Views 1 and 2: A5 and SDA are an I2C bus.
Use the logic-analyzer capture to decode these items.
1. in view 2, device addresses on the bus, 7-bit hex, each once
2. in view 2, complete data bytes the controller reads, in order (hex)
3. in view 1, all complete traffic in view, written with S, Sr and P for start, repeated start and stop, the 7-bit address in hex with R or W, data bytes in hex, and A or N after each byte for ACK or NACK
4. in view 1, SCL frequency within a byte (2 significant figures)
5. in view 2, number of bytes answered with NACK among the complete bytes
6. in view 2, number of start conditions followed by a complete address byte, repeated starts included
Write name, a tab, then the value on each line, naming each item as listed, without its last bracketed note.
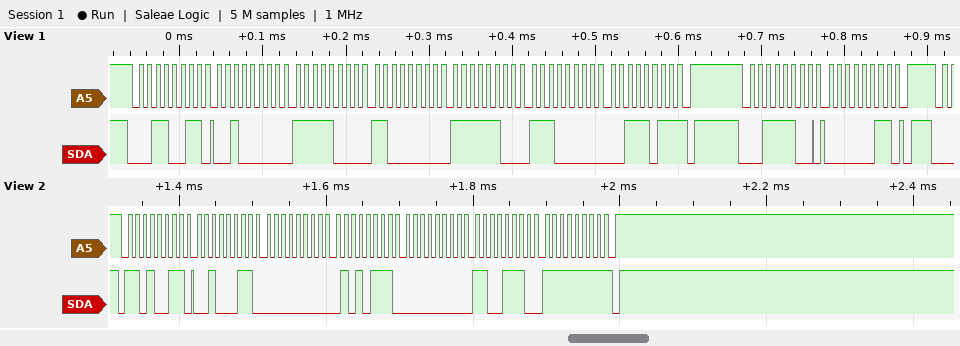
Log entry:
in view 2, device addresses on the bus, 7-bit hex, each once	0x69
in view 2, complete data bytes the controller reads, in order	23 00 57 00 CE FF
in view 1, all complete traffic in view, written with S, Sr and P for start, repeated start and stop, the 7-bit address in hex with R or W, data bytes in hex, and A or N after each byte for ACK or NACK	S 19R A 20 A F8 A C0 A FC A E0 A 3B N P S 1EW A 03 A P
in view 1, SCL frequency within a byte	100 kHz
in view 2, number of bytes answered with NACK among the complete bytes	1
in view 2, number of start conditions followed by a complete address byte, repeated starts included	1
